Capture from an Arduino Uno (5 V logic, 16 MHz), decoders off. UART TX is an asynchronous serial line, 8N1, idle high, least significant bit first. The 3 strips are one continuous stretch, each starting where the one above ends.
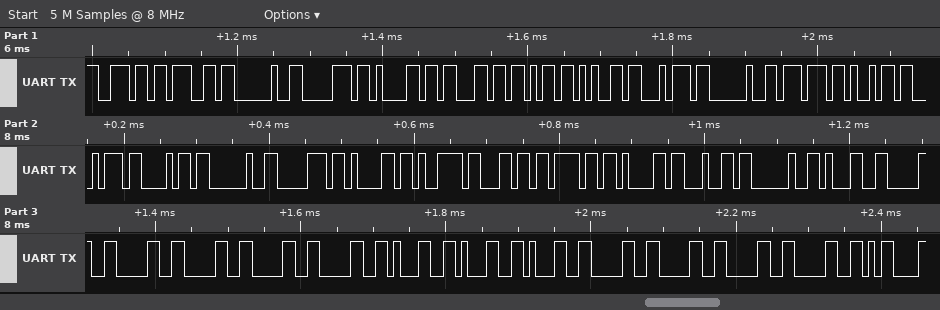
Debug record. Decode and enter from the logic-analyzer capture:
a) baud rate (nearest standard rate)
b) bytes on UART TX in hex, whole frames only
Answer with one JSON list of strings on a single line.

["115200 baud", "6E 67 20 70 61 63 6B 65 74 20 77 69 74 68 20 70 61 79 6C 6F 61 64 20 31 30 30 30 30 30 31 31 31 30 30 30 30 0D"]
